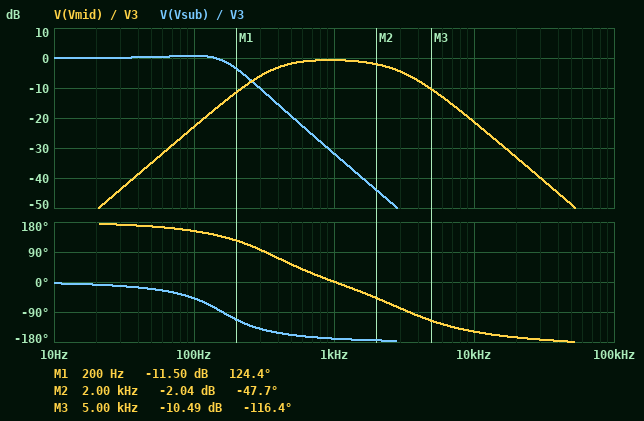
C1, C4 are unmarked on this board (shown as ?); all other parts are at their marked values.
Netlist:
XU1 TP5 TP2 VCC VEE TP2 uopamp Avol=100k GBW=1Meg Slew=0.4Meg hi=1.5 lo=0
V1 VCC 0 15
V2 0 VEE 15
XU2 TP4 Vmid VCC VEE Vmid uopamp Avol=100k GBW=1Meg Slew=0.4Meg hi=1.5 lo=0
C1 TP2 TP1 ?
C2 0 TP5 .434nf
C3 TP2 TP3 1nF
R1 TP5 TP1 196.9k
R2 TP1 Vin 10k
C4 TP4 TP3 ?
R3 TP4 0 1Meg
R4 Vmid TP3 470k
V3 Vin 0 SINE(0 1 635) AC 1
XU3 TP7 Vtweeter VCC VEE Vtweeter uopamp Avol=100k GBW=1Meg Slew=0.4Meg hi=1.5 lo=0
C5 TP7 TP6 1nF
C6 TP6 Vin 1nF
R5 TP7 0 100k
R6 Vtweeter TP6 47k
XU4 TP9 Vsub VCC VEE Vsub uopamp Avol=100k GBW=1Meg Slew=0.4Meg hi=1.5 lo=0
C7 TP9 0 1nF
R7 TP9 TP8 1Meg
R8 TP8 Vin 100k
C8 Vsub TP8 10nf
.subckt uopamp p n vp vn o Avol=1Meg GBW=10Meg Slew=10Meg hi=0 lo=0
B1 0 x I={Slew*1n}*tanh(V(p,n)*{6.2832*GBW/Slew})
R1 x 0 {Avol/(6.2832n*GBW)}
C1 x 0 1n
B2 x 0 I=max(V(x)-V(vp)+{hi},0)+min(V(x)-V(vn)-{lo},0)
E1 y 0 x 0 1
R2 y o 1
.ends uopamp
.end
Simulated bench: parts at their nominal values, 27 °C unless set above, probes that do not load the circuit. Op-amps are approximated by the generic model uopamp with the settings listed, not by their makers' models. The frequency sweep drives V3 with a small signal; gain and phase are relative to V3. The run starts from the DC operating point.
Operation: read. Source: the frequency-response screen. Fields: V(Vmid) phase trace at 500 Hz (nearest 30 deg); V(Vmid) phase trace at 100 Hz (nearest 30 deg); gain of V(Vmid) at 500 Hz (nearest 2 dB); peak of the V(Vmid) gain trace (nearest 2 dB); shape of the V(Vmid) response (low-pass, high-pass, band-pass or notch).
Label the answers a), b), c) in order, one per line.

a) 60 deg
b) 150 deg
c) -2 dB
d) 0 dB
e) band-pass
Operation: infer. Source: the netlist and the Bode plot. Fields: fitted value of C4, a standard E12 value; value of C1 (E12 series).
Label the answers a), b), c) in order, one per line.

a) 390 pF
b) 3.3 nF
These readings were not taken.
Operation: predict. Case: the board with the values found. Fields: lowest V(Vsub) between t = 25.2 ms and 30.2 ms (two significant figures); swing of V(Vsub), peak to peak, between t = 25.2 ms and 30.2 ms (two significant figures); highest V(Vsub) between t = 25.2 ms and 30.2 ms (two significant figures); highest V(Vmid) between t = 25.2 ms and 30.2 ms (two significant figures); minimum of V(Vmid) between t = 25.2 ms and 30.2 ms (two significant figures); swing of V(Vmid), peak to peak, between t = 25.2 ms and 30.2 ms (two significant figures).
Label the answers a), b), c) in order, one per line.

a) -64 mV
b) 130 mV
c) 64 mV
d) 880 mV
e) -880 mV
f) 1.8 V
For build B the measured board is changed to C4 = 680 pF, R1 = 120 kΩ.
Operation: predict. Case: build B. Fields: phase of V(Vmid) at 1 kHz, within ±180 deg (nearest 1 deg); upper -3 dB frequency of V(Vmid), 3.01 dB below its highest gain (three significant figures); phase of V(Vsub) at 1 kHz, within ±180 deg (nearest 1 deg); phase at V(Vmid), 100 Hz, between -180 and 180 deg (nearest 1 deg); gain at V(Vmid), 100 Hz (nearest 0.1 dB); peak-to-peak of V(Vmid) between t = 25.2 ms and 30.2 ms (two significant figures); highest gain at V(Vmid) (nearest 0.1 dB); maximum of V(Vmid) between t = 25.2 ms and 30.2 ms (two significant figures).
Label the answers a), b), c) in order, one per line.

a) 2 deg
b) 3.97 kHz
c) -170 deg
d) 148 deg
e) -18.0 dB
f) 2.0 V
g) 0 dB
h) 990 mV
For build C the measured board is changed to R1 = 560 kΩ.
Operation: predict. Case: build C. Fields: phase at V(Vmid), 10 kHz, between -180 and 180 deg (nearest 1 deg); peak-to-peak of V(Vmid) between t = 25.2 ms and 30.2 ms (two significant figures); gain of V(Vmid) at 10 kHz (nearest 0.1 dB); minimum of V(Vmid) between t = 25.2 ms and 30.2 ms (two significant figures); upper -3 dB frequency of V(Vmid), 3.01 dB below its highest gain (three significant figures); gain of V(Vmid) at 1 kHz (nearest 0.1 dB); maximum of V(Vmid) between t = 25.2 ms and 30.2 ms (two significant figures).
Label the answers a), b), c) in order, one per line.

a) -151 deg
b) 1.4 V
c) -30.7 dB
d) -680 mV
e) 1.25 kHz
f) -4.9 dB
g) 680 mV
